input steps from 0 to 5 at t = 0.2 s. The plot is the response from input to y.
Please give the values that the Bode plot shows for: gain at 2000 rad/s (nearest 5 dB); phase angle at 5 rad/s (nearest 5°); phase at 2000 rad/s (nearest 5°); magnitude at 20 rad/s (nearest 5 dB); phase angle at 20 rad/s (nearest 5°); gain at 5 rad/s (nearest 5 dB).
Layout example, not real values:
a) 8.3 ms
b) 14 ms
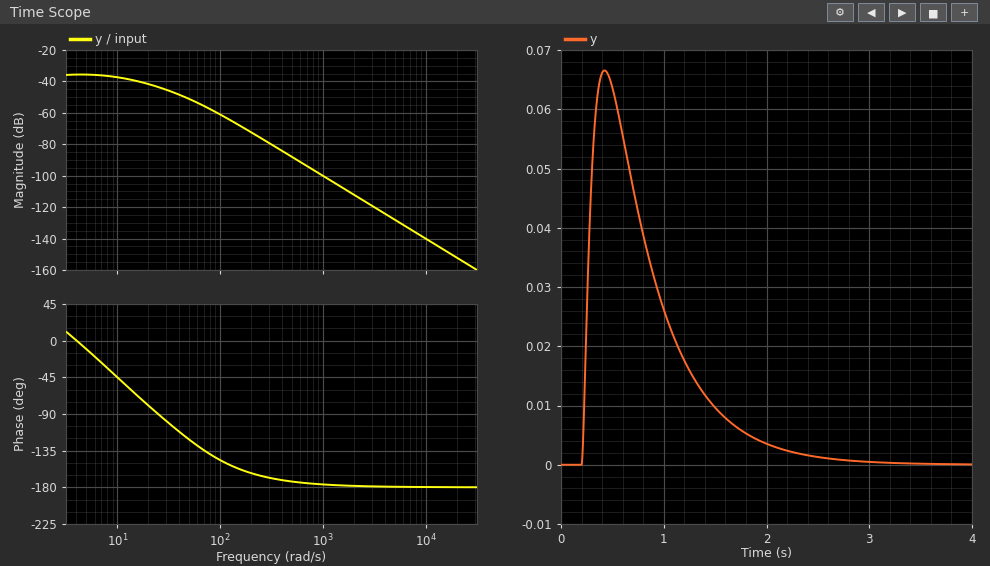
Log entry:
a) -110 dB
b) -10°
c) -180°
d) -40 dB
e) -80°
f) -35 dB
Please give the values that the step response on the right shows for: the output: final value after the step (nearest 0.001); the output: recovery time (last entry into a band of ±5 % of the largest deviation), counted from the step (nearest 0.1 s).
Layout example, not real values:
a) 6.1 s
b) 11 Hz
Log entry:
a) 0.000
b) 1.8 s
